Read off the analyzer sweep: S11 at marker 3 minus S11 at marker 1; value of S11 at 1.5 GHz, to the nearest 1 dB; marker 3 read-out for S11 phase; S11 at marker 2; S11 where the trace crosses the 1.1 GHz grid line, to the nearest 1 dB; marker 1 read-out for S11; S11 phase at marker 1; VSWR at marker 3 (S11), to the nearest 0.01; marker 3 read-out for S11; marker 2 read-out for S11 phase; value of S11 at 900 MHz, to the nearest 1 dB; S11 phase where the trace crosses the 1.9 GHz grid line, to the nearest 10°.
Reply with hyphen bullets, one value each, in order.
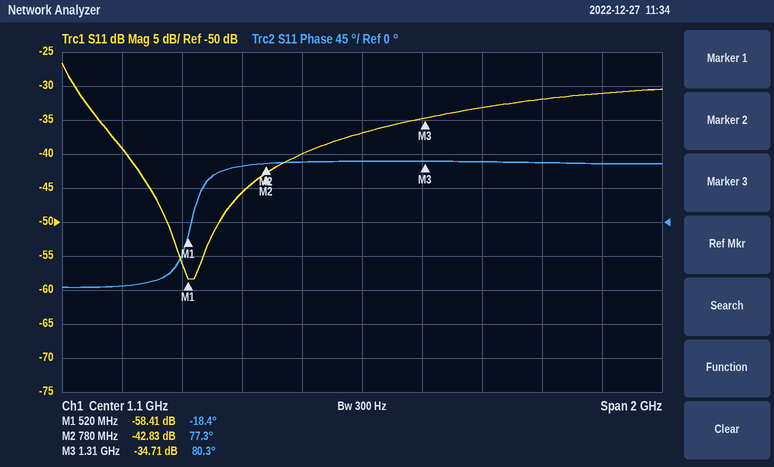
- 23.70 dB
- -33 dB
- 80.3°
- -42.83 dB
- -37 dB
- -58.41 dB
- -18.4°
- 1.04
- -34.71 dB
- 77.3°
- -40 dB
- 80°
